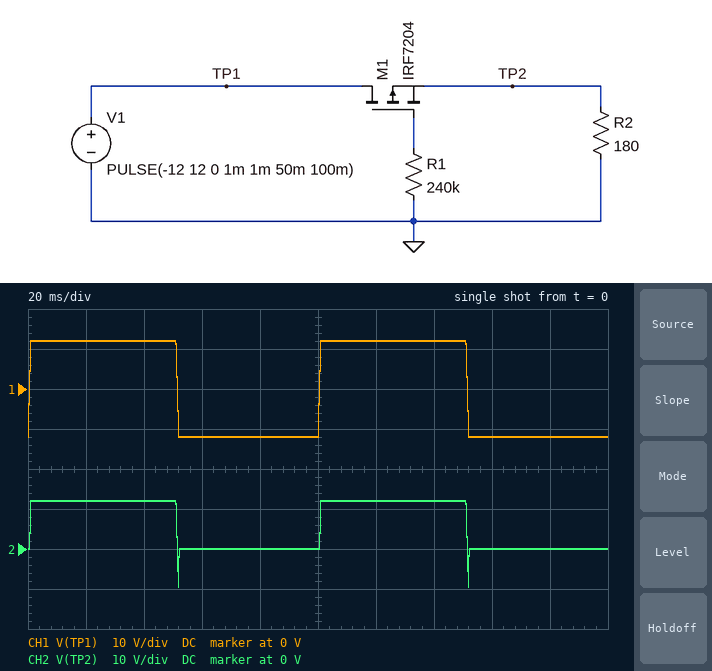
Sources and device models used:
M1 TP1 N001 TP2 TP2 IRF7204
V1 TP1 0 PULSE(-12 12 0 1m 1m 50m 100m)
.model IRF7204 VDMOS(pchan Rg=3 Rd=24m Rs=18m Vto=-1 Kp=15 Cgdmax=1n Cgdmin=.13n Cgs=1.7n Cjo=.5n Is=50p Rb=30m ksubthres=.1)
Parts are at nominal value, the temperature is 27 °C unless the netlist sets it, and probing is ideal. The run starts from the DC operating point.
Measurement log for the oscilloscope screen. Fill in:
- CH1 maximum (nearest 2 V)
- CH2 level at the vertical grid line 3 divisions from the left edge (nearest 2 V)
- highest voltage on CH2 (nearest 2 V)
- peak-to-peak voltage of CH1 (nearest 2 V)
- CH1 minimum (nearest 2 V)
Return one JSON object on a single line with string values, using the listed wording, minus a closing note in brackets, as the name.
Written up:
{"CH1 maximum": "12 V", "CH2 level at the vertical grid line 3 divisions from the left edge": "0 V", "highest voltage on CH2": "12 V", "peak-to-peak voltage of CH1": "24 V", "CH1 minimum": "-12 V"}
